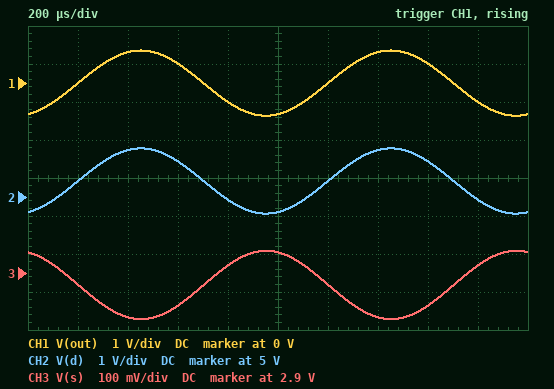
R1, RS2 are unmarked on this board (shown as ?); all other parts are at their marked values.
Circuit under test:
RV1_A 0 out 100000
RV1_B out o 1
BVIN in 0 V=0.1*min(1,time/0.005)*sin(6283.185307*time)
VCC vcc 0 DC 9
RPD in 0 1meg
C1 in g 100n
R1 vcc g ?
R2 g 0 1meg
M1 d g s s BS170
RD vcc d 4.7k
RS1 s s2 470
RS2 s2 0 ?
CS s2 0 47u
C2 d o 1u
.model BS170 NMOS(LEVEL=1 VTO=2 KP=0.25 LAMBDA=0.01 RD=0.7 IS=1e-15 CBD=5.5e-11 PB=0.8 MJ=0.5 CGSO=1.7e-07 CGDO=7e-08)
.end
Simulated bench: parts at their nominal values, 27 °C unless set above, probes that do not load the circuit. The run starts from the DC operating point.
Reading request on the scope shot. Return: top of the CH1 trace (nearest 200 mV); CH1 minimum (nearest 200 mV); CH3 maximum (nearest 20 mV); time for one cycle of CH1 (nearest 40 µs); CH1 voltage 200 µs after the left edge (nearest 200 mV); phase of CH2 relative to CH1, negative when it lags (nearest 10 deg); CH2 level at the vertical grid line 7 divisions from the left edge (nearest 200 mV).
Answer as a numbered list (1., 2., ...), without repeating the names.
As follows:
1. 800 mV
2. -800 mV
3. 2.96 V
4. 1.00 ms
5. 0 V
6. 0 deg
7. 6.2 V
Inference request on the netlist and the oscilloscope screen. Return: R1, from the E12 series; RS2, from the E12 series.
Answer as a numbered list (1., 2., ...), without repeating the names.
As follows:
1. 820 kΩ
2. 3.3 kΩ
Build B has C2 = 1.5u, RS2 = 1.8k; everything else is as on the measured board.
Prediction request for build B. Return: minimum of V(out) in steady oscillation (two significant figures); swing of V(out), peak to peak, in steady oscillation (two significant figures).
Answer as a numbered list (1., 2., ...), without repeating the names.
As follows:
1. -270 mV
2. 930 mV
